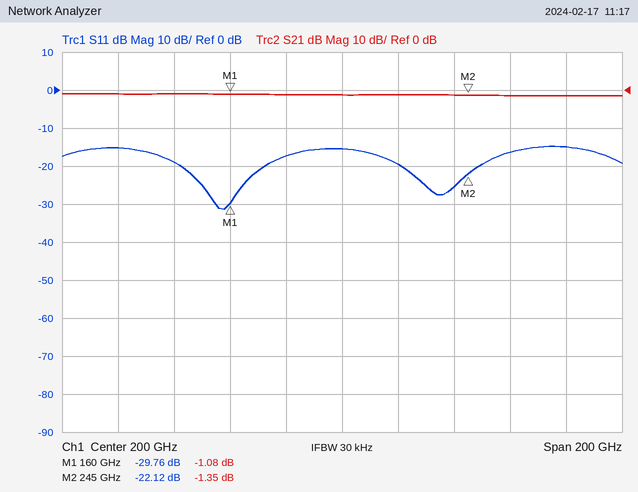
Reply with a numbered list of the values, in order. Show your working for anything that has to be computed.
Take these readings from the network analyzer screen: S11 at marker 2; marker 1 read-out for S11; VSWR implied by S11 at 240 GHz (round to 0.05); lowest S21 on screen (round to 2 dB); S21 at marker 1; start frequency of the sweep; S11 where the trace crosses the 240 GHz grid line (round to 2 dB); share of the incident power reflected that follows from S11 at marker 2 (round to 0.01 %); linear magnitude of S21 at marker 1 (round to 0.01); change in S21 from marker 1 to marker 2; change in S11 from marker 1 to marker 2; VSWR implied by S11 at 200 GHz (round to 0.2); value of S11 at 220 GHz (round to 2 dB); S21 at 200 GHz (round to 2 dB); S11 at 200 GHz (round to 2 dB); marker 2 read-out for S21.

1. -22.12 dB
2. -29.76 dB
3. |Γ| = 10^(-26/20) = 0.0501; VSWR = (1 + 0.0501)/(1 − 0.0501) ≈ 1.11, so 1.10 to the nearest 0.05
4. -2 dB
5. -1.08 dB
6. 100 GHz
7. -26 dB
8. 10^(-22.12/10) ≈ 0.61 %
9. 10^(-1.08/20) ≈ 0.88
10. -1.35 − (-1.08) = -0.27 dB
11. -22.12 − (-29.76) = 7.64 dB
12. |Γ| = 10^(-16/20) = 0.1585; VSWR = (1 + 0.1585)/(1 − 0.1585) ≈ 1.4
13. -20 dB
14. -2 dB
15. -16 dB
16. -1.35 dB
